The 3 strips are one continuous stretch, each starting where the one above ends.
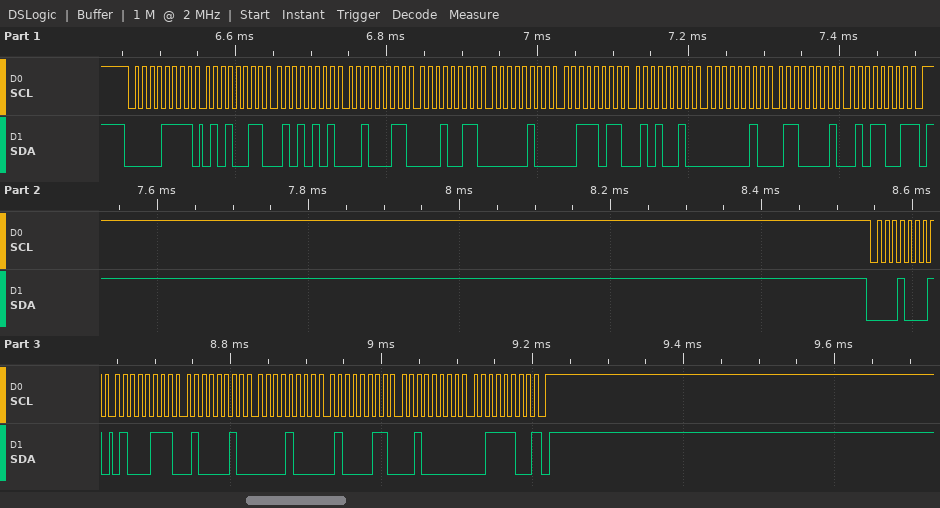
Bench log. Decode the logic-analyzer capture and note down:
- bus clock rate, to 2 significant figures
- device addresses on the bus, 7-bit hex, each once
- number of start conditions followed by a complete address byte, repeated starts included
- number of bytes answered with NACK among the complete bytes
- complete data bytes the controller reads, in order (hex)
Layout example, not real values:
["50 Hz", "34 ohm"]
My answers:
["100 kHz", "0x07 0x08", "2", "2", "53 55 23 13 04 3B 52 02 61 59 47 42 08 43 20 3C"]
